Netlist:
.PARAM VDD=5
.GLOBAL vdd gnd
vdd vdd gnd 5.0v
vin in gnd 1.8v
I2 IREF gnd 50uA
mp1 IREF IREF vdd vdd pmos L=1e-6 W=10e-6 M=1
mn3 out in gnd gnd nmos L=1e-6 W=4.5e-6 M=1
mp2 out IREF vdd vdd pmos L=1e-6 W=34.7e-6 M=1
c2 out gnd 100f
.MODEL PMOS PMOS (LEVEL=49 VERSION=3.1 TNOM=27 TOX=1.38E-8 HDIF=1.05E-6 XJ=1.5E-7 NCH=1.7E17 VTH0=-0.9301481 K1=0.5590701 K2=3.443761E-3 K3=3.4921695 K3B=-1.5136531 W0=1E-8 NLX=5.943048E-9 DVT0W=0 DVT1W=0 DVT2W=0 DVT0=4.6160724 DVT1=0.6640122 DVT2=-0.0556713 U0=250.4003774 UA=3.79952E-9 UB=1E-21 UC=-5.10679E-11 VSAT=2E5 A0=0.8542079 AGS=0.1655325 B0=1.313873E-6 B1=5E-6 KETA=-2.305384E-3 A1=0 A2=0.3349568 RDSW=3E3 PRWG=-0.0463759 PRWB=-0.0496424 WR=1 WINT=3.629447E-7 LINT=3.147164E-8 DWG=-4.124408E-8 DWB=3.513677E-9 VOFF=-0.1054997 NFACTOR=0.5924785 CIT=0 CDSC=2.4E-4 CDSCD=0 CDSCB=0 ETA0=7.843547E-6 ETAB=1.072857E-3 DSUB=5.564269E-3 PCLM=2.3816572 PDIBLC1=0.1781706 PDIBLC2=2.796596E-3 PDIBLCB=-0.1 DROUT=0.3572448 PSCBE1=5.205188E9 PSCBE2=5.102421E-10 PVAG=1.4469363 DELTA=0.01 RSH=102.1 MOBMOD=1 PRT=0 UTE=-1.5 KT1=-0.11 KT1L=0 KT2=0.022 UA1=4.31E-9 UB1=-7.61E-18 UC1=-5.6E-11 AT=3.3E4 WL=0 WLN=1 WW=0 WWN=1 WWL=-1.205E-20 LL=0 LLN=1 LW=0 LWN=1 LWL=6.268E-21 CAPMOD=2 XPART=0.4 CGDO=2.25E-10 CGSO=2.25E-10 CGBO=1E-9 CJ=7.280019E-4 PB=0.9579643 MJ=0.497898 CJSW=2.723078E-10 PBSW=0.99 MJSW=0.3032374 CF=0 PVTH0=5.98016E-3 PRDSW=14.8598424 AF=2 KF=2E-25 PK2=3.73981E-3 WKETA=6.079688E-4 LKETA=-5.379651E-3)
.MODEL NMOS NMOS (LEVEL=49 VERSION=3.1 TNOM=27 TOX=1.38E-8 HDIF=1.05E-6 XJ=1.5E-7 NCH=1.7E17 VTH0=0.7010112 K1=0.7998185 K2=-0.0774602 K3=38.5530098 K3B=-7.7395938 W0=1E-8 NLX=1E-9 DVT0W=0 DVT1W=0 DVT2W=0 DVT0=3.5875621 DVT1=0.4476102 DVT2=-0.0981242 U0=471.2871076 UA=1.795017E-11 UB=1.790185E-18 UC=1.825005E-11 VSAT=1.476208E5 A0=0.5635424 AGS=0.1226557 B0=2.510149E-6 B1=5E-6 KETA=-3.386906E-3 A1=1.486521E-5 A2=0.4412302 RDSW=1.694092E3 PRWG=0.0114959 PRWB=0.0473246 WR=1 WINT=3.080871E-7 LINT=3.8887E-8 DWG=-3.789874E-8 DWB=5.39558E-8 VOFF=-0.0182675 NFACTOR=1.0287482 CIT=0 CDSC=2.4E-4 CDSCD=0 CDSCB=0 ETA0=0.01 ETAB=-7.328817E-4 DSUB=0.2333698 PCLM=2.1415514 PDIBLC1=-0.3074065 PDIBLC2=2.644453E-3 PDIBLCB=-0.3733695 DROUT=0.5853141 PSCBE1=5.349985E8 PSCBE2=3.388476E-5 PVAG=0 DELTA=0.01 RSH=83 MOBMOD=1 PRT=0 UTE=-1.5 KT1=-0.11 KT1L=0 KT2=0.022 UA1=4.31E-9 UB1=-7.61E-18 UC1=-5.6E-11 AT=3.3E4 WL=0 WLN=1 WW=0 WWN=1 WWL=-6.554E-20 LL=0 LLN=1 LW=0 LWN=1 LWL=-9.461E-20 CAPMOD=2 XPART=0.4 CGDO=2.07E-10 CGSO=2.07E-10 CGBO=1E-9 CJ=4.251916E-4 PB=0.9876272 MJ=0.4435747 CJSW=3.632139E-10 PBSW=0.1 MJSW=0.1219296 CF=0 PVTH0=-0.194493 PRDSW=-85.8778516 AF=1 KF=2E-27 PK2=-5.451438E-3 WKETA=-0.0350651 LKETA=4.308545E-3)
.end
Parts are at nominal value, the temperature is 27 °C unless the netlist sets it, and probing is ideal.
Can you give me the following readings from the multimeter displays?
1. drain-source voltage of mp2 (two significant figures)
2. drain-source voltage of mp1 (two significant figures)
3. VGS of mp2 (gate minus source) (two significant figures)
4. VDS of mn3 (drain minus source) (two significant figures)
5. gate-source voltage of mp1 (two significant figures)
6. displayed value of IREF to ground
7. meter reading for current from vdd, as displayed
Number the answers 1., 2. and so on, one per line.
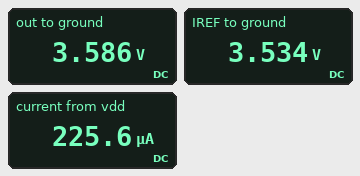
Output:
1. -1.4 V
2. -1.5 V
3. -1.5 V
4. 3.6 V
5. -1.5 V
6. 3.534 V
7. 225.6 µA
